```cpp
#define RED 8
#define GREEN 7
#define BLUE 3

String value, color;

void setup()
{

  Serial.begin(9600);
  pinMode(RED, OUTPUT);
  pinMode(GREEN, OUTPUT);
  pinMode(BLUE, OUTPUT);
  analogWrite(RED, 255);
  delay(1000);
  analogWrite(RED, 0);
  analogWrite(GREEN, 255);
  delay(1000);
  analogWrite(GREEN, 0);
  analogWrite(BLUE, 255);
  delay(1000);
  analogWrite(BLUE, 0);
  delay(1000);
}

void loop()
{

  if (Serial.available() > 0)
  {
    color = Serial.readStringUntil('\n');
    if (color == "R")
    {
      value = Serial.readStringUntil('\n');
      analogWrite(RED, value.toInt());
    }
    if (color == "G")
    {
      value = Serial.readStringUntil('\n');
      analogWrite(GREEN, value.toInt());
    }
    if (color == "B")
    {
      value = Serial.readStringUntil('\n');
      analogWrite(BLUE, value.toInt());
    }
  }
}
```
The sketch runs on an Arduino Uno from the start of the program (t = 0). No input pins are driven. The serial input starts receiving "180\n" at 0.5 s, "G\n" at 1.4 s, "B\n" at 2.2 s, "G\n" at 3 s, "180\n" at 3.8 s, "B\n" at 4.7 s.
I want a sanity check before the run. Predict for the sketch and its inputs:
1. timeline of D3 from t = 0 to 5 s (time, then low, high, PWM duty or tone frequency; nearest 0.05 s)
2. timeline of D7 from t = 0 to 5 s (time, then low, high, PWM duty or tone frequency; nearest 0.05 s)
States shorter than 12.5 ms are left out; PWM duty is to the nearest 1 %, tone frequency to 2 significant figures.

0 s low; 2 s high; 3 s low
0 s low; 1 s high; 2 s low; 4 s high
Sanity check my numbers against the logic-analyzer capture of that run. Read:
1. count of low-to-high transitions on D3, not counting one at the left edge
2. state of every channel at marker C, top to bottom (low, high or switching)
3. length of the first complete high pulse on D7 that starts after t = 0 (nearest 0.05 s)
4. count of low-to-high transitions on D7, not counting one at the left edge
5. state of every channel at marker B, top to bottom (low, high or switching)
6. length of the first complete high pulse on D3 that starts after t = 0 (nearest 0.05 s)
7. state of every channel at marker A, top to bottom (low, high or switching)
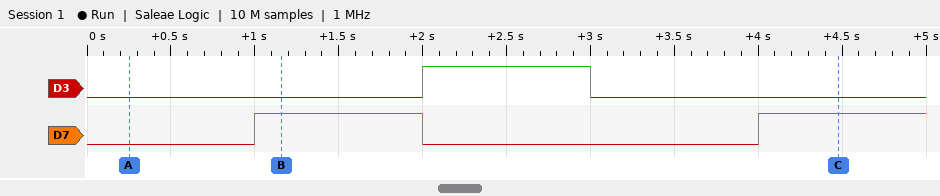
1
D3 low, D7 high
1.00 s
2
D3 low, D7 high
1.00 s
D3 low, D7 low
